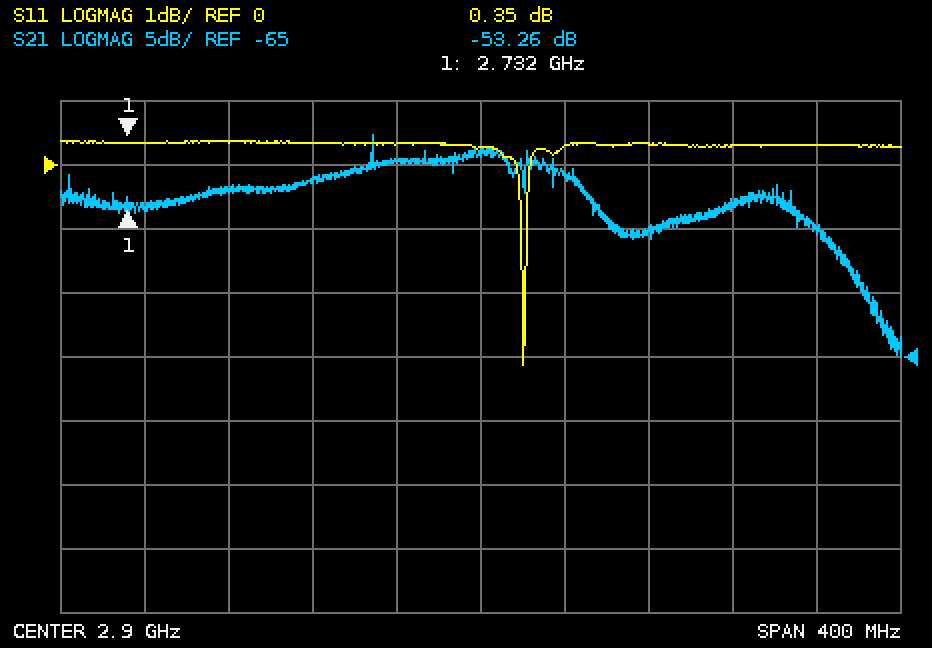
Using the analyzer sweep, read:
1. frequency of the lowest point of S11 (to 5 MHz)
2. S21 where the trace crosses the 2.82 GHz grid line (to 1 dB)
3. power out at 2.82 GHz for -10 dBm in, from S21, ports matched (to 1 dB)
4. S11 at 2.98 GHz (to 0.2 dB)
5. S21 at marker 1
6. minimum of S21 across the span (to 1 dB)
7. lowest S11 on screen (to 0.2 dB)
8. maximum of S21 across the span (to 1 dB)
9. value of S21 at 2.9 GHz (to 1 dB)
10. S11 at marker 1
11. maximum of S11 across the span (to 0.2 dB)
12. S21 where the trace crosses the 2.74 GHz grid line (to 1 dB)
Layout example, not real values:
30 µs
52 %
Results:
2.920 GHz
-51 dB
-61 dBm
0.4 dB
-53.26 dB
-65 dB
-3.2 dB
-48 dB
-49 dB
0.35 dB
0.4 dB
-53 dB
